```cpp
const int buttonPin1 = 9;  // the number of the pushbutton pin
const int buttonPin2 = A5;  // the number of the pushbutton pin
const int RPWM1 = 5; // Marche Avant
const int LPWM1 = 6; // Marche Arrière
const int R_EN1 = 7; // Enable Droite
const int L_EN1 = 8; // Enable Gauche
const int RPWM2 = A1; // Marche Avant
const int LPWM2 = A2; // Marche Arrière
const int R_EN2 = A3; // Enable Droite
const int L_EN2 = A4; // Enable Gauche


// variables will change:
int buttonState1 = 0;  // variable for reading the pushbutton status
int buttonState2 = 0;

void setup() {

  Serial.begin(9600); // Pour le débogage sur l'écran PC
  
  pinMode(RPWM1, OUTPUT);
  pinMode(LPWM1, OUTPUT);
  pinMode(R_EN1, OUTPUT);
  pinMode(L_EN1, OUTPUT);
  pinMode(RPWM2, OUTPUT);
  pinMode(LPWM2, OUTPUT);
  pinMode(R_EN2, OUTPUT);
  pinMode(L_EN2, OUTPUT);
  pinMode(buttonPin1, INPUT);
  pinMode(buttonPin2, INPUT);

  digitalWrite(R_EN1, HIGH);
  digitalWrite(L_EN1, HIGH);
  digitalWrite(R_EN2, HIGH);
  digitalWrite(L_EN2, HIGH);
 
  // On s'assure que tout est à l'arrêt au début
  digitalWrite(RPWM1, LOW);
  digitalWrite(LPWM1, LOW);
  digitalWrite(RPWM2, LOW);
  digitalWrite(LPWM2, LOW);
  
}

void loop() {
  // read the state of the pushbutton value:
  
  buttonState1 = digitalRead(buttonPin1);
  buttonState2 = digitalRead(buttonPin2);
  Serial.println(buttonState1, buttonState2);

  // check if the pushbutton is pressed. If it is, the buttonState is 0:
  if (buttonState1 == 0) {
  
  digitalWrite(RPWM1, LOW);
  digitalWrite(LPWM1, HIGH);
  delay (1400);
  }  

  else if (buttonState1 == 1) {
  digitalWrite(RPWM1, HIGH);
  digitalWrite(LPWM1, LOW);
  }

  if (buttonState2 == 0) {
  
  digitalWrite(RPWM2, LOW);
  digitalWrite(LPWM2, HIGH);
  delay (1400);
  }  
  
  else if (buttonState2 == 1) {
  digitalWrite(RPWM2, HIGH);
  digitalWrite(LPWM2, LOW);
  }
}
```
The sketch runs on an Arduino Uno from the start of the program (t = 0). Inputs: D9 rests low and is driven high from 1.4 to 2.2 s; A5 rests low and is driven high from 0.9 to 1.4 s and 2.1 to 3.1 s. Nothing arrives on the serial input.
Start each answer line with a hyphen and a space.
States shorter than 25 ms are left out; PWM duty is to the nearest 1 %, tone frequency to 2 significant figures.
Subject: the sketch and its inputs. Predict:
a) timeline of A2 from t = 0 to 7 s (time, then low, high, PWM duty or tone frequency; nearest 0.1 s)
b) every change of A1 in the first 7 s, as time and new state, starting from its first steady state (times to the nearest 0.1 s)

- 0 s low; 1.4 s high; 4.2 s low; 5.6 s high
- 0 s low; 4.2 s high; 5.6 s low
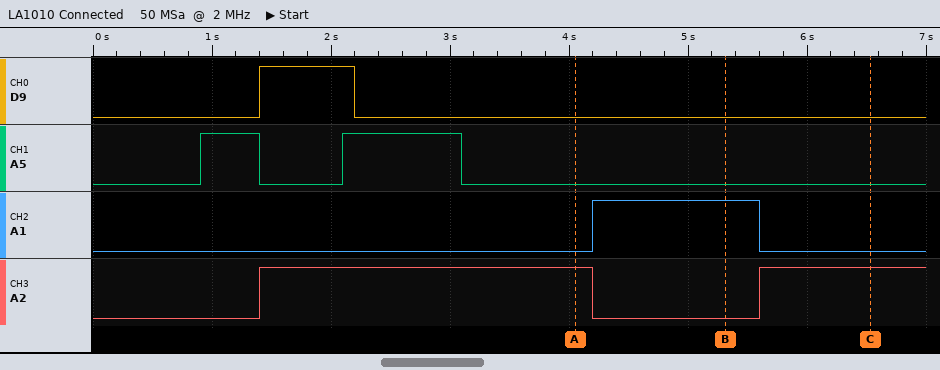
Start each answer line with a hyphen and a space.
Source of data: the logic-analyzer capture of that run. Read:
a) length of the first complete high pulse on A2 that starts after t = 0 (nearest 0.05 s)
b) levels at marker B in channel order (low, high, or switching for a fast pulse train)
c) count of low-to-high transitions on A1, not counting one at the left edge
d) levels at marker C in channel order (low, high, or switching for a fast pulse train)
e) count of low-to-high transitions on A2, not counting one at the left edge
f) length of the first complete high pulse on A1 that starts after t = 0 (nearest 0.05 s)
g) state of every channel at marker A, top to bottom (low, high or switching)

- 2.80 s
- D9 low, A5 low, A1 high, A2 low
- 1
- D9 low, A5 low, A1 low, A2 high
- 2
- 1.40 s
- D9 low, A5 low, A1 low, A2 high
